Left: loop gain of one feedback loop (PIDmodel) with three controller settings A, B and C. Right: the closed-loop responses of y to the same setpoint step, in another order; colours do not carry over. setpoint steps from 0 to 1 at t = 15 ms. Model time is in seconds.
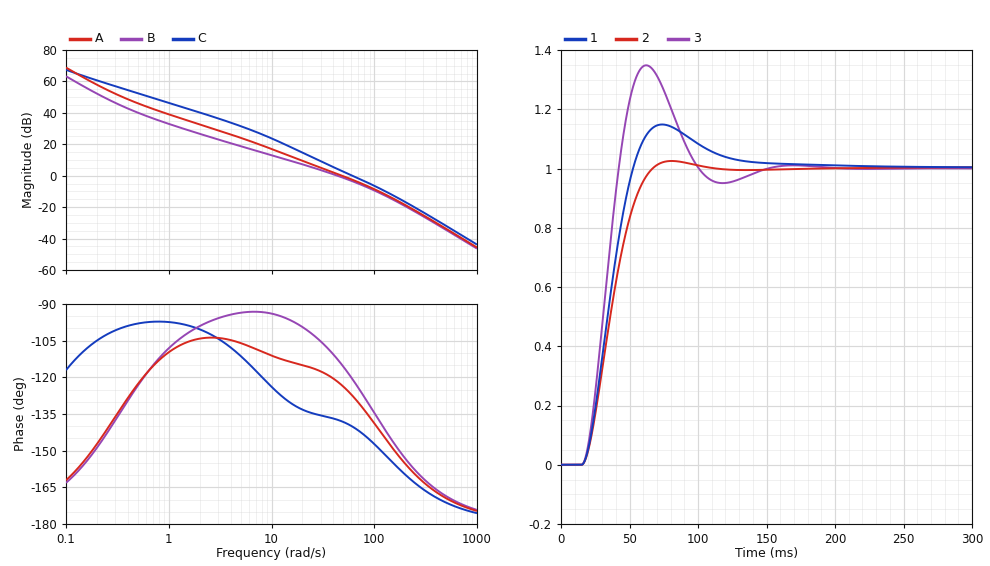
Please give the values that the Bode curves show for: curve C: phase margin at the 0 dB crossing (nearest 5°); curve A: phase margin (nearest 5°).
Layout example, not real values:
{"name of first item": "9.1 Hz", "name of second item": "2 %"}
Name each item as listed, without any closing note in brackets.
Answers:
{"curve C: phase margin at the 0 dB crossing": "40°", "curve A: phase margin": "55°"}
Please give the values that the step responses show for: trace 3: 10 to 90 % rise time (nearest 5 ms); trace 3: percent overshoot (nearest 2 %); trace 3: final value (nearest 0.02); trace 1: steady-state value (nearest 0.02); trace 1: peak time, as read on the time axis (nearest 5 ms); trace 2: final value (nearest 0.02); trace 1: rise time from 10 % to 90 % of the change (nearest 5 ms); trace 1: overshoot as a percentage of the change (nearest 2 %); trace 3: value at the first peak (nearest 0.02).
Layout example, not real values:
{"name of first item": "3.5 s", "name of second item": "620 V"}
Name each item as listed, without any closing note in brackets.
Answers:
{"trace 3: 10 to 90 % rise time": "20 ms", "trace 3: percent overshoot": "34 %", "trace 3: final value": "1.00", "trace 1: steady-state value": "1.00", "trace 1: peak time, as read on the time axis": "75 ms", "trace 2: final value": "1.00", "trace 1: rise time from 10 % to 90 % of the change": "25 ms", "trace 1: overshoot as a percentage of the change": "14 %", "trace 3: value at the first peak": "1.34"}
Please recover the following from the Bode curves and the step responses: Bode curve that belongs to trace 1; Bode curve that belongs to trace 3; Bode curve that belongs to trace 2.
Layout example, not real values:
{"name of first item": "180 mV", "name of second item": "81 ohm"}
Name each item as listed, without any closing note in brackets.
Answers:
{"Bode curve that belongs to trace 1": "A", "Bode curve that belongs to trace 3": "C", "Bode curve that belongs to trace 2": "B"}
